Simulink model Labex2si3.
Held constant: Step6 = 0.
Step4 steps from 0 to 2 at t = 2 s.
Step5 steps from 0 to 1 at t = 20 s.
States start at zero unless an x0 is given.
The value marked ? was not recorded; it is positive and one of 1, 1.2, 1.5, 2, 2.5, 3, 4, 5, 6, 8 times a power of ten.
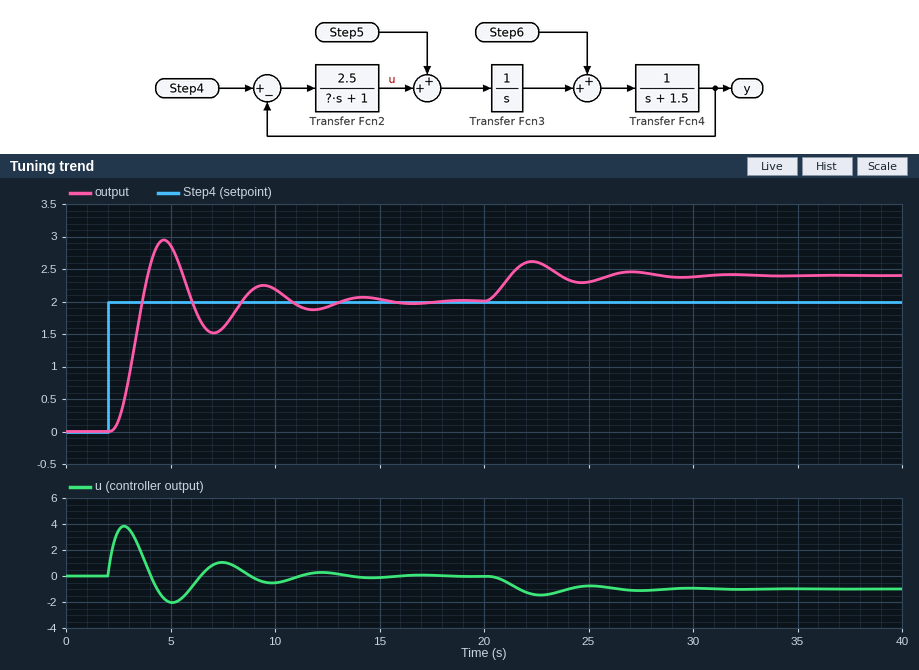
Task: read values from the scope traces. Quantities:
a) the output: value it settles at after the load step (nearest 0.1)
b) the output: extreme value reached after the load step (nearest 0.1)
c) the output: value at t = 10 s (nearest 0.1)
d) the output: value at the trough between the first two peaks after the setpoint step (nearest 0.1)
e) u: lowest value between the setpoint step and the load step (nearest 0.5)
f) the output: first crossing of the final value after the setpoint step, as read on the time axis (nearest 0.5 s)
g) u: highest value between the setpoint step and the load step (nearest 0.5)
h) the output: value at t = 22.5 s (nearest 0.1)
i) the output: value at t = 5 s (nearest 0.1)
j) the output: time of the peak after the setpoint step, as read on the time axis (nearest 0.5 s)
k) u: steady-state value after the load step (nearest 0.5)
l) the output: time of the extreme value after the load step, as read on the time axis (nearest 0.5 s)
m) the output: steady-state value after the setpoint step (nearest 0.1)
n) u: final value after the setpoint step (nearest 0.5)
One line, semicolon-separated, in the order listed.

2.4; 2.6; 2.2; 1.5; -2.0; 3.5 s; 4.0; 2.6; 2.9; 4.5 s; -1.0; 22.5 s; 2.0; 0.0
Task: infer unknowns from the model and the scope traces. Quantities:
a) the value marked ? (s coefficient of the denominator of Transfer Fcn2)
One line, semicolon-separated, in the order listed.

0.4
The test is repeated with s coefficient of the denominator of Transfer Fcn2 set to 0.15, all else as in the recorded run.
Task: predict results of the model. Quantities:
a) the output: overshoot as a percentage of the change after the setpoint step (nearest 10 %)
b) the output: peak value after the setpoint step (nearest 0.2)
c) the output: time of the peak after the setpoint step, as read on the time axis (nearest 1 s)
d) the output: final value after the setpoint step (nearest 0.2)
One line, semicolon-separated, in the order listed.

30 %; 2.6; 4 s; 2.0
